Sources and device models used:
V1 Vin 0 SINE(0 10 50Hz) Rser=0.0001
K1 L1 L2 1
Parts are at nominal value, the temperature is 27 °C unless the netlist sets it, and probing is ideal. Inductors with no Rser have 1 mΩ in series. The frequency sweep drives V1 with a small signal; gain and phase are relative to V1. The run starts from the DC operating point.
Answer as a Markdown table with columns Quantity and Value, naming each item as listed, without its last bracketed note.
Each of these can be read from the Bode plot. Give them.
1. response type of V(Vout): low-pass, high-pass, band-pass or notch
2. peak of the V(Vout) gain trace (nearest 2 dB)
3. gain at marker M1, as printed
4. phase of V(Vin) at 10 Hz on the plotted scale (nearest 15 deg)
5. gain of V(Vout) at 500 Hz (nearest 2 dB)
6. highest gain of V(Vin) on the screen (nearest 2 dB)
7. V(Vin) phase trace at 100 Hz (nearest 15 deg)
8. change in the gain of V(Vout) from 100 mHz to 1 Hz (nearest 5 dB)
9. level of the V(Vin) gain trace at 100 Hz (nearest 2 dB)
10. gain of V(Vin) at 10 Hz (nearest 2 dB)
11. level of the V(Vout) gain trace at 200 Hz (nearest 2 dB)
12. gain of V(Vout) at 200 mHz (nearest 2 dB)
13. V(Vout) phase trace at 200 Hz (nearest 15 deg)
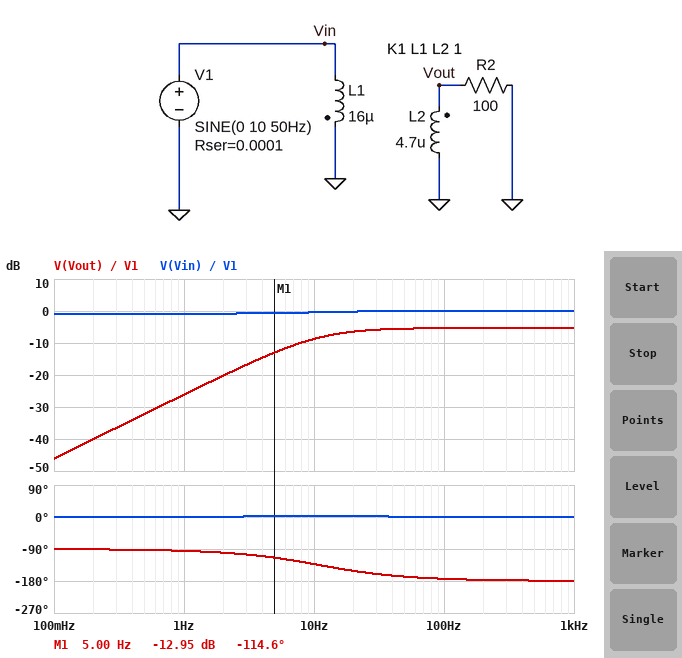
| Quantity | Value |
|---|---|
| response type of V(Vout): low-pass, high-pass, band-pass or notch | high-pass |
| peak of the V(Vout) gain trace | -6 dB |
| gain at marker M1, as printed | -12.95 dB |
| phase of V(Vin) at 10 Hz on the plotted scale | 0 deg |
| gain of V(Vout) at 500 Hz | -6 dB |
| highest gain of V(Vin) on the screen | 0 dB |
| V(Vin) phase trace at 100 Hz | 0 deg |
| change in the gain of V(Vout) from 100 mHz to 1 Hz | 20 dB |
| level of the V(Vin) gain trace at 100 Hz | 0 dB |
| gain of V(Vin) at 10 Hz | 0 dB |
| level of the V(Vout) gain trace at 200 Hz | -6 dB |
| gain of V(Vout) at 200 mHz | -40 dB |
| V(Vout) phase trace at 200 Hz | -180 deg |
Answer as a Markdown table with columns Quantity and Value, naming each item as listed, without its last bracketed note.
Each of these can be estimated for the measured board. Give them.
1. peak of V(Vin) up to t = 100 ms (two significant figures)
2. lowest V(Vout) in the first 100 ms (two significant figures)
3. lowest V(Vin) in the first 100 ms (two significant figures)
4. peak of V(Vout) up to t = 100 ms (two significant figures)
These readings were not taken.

| Quantity | Value |
|---|---|
| peak of V(Vin) up to t = 100 ms | 10 V |
| lowest V(Vout) in the first 100 ms | -5.3 V |
| lowest V(Vin) in the first 100 ms | -10 V |
| peak of V(Vout) up to t = 100 ms | 5.7 V |
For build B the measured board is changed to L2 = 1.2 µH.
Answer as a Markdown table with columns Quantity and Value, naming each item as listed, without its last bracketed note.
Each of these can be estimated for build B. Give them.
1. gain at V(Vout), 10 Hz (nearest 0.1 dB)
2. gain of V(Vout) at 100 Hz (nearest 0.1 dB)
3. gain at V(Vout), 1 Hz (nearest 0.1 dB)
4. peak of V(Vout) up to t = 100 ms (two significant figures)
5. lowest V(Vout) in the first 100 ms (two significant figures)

| Quantity | Value |
|---|---|
| gain at V(Vout), 10 Hz | -14.7 dB |
| gain of V(Vout) at 100 Hz | -11.3 dB |
| gain at V(Vout), 1 Hz | -32.1 dB |
| peak of V(Vout) up to t = 100 ms | 2.9 V |
| lowest V(Vout) in the first 100 ms | -2.7 V |
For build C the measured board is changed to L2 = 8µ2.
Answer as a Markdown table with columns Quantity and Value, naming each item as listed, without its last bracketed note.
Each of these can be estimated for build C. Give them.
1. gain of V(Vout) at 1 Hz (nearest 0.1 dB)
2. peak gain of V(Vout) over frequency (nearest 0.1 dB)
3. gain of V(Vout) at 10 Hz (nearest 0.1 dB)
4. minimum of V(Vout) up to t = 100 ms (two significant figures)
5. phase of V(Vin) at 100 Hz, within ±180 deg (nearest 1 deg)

| Quantity | Value |
|---|---|
| gain of V(Vout) at 1 Hz | -23.7 dB |
| peak gain of V(Vout) over frequency | -2.9 dB |
| gain of V(Vout) at 10 Hz | -6.3 dB |
| minimum of V(Vout) up to t = 100 ms | -7.0 V |
| phase of V(Vin) at 100 Hz, within ±180 deg | 1 deg |
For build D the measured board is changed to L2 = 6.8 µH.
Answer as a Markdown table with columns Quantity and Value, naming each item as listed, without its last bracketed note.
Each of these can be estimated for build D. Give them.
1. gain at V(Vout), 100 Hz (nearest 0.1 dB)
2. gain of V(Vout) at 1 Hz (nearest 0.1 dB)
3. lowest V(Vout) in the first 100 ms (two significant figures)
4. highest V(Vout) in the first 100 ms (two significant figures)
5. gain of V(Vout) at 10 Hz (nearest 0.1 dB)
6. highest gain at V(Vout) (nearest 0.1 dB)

| Quantity | Value |
|---|---|
| gain at V(Vout), 100 Hz | -3.8 dB |
| gain of V(Vout) at 1 Hz | -24.5 dB |
| lowest V(Vout) in the first 100 ms | -6.4 V |
| highest V(Vout) in the first 100 ms | 6.9 V |
| gain of V(Vout) at 10 Hz | -7.1 dB |
| highest gain at V(Vout) | -3.7 dB |
